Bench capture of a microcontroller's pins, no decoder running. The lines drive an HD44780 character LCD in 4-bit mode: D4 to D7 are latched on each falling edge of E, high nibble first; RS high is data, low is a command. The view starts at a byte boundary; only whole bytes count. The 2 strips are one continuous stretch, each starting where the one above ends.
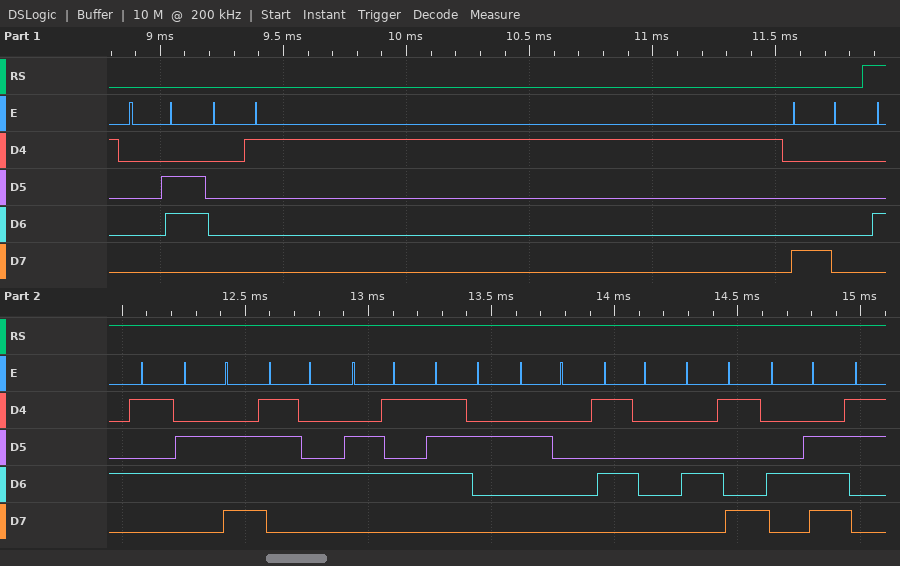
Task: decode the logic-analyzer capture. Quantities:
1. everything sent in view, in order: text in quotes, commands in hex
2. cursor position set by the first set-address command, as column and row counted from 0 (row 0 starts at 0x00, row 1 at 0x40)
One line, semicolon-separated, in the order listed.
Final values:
0x06 0x01 0x80 "Enter PIN"; column 0, row 0
